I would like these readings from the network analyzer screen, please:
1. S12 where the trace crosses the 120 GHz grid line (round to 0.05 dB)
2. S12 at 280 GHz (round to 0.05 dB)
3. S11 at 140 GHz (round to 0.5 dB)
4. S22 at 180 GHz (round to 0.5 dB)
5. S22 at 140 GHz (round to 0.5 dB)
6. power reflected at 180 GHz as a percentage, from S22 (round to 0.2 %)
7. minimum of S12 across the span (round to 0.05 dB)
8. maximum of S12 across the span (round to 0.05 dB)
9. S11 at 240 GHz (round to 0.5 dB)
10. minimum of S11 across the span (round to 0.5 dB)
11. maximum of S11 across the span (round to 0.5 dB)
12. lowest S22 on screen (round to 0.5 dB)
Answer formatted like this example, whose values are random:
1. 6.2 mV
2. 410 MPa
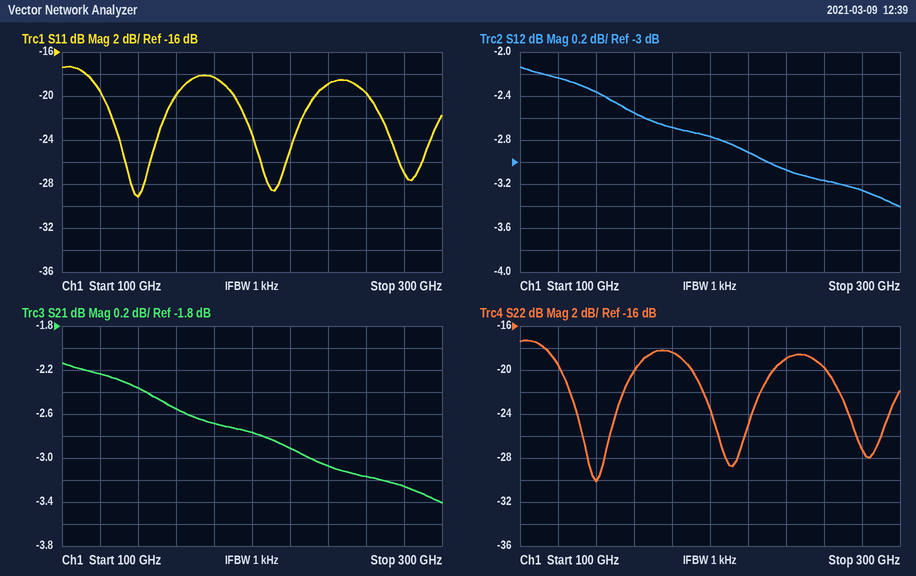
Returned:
1. -2.25 dB
2. -3.25 dB
3. -29.0 dB
4. -18.5 dB
5. -30.0 dB
6. 1.4 %
7. -3.40 dB
8. -2.15 dB
9. -19.0 dB
10. -29.0 dB
11. -17.5 dB
12. -30.0 dB
